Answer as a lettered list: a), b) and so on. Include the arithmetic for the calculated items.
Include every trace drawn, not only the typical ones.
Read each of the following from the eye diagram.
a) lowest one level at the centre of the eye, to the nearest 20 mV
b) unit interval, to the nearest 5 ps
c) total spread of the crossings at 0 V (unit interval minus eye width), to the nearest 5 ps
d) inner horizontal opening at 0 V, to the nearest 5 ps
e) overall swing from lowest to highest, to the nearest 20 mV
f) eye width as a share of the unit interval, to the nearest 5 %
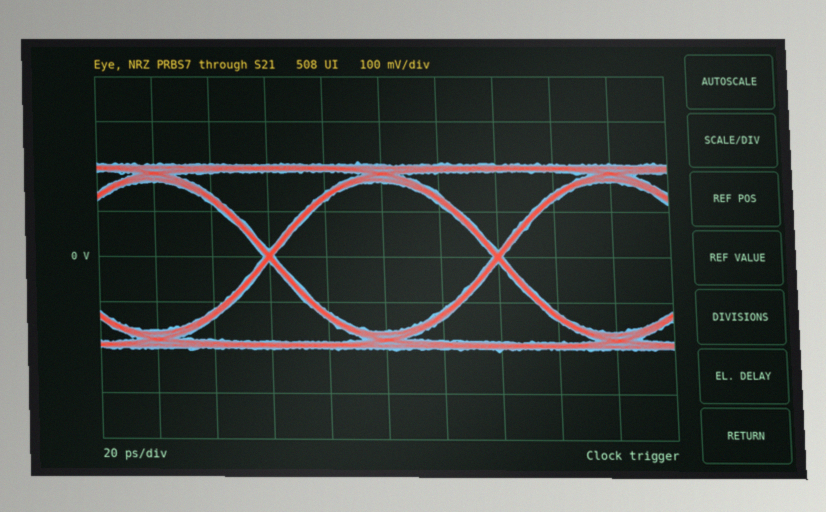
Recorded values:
a) 160 mV
b) 80 ps
c) 5 ps
d) 75 ps
e) 420 mV
f) 75 ps / 80 ps ≈ 93.8 %, so 95 % to the nearest 5 %
